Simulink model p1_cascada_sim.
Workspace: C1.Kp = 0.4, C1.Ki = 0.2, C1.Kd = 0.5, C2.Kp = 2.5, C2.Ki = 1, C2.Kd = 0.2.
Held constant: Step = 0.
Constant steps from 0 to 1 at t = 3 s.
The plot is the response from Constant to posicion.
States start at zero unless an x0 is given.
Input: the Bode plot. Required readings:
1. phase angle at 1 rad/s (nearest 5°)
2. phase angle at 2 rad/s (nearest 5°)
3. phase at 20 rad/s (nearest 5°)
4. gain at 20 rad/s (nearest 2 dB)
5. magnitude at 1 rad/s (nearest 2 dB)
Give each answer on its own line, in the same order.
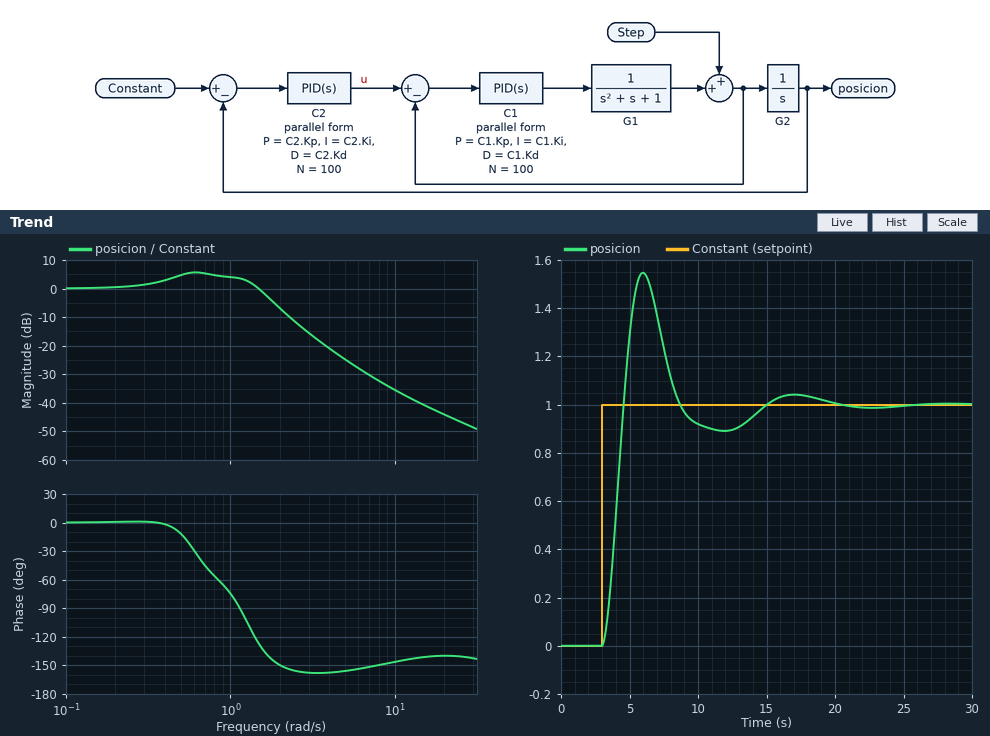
-75°
-150°
-140°
-44 dB
4 dB
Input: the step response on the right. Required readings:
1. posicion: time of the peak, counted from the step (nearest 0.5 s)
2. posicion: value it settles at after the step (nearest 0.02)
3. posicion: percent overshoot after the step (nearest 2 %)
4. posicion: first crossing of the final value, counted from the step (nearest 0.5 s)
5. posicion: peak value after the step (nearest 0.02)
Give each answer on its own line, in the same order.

3.0 s
1.00
54 %
1.5 s
1.54
